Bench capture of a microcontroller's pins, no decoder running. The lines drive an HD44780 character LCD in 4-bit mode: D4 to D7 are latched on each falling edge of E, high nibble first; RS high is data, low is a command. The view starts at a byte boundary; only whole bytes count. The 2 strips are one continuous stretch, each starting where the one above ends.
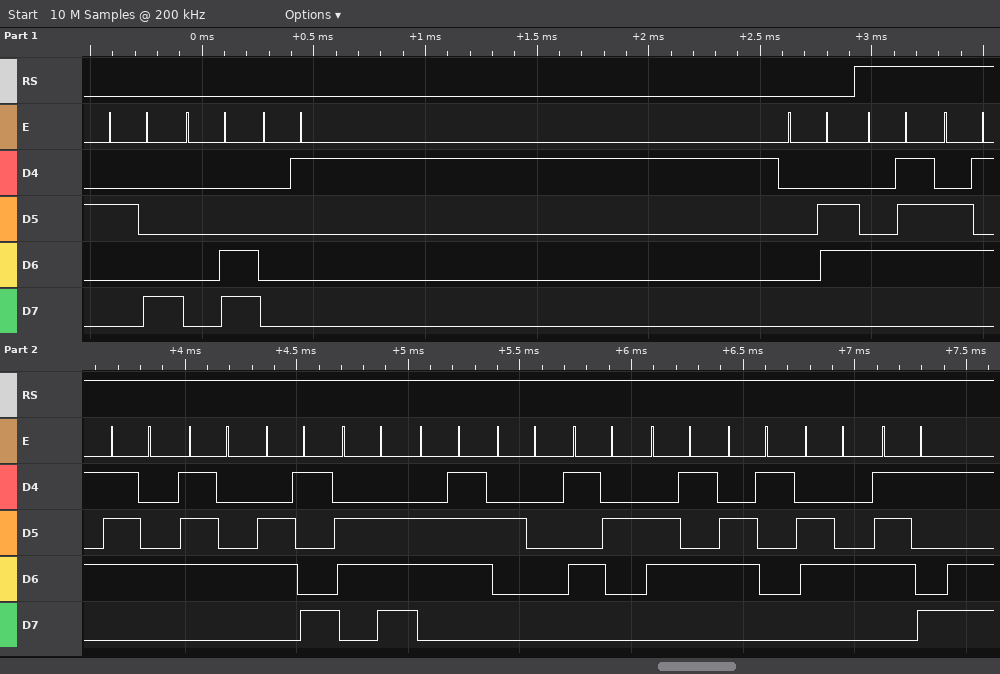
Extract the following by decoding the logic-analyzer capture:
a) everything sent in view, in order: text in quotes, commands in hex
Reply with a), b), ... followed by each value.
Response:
a) 0x28 0x0C 0x01 0x06 "Getting Ready"
